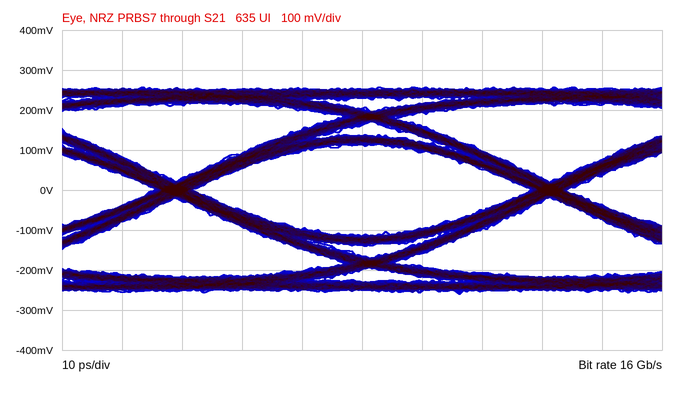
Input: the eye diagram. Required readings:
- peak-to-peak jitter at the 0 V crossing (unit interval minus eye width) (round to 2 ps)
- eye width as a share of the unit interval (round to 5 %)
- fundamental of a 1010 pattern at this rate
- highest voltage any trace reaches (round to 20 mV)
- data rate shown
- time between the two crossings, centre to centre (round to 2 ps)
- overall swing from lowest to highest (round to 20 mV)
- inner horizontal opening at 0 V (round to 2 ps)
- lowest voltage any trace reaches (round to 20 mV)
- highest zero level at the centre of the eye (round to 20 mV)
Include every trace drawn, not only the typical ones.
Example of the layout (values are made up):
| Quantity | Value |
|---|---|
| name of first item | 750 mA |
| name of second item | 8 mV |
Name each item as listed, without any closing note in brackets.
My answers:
| Quantity | Value |
|---|---|
| peak-to-peak jitter at the 0 V crossing (unit interval minus eye width) | 6 ps |
| eye width as a share of the unit interval | 90 % |
| fundamental of a 1010 pattern at this rate | 8 GHz |
| highest voltage any trace reaches | 260 mV |
| data rate shown | 16 Gb/s |
| time between the two crossings, centre to centre | 62 ps |
| overall swing from lowest to highest | 520 mV |
| inner horizontal opening at 0 V | 56 ps |
| lowest voltage any trace reaches | -260 mV |
| highest zero level at the centre of the eye | -120 mV |
